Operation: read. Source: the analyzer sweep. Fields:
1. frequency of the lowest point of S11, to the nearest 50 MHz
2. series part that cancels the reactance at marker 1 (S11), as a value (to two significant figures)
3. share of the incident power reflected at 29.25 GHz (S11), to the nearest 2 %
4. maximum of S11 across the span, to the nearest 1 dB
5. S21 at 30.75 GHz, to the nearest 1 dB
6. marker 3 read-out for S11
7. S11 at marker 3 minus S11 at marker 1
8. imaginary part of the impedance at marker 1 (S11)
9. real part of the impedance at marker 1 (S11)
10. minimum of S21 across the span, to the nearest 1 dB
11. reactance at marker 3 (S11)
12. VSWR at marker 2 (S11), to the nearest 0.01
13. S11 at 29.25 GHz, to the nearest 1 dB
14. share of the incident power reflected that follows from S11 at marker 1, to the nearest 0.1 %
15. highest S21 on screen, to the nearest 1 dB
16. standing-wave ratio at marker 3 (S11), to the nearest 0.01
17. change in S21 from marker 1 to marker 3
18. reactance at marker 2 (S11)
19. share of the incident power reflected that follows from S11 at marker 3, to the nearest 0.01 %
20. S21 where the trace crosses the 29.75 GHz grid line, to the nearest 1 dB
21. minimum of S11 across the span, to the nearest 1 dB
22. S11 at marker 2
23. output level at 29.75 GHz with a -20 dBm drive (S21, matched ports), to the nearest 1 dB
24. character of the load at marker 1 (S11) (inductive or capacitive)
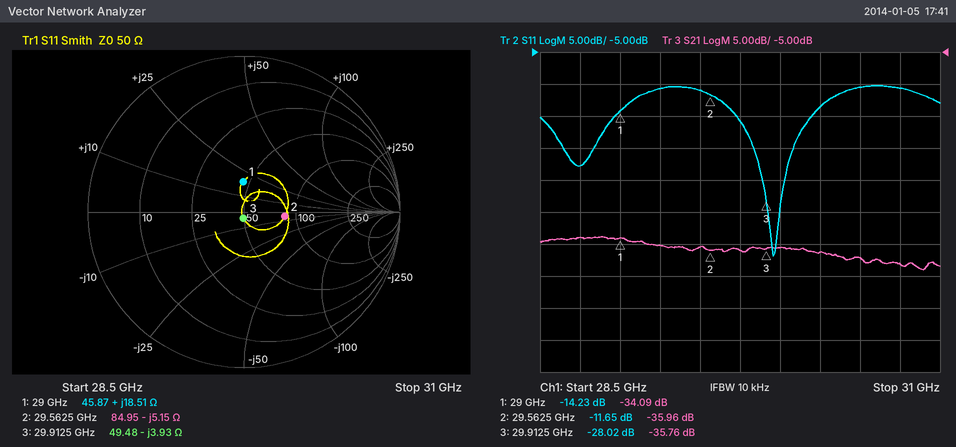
29.95 GHz
300 fF
8 %
-10 dB
-38 dB
-28.02 dB
-13.79 dB
+18.51 Ω
45.87 Ω
-39 dB
-3.93 Ω
1.71
-11 dB
3.8 %
-34 dB
1.08
-1.67 dB
-5.15 Ω
0.16 %
-36 dB
-37 dB
-11.65 dB
-56 dBm
inductive
